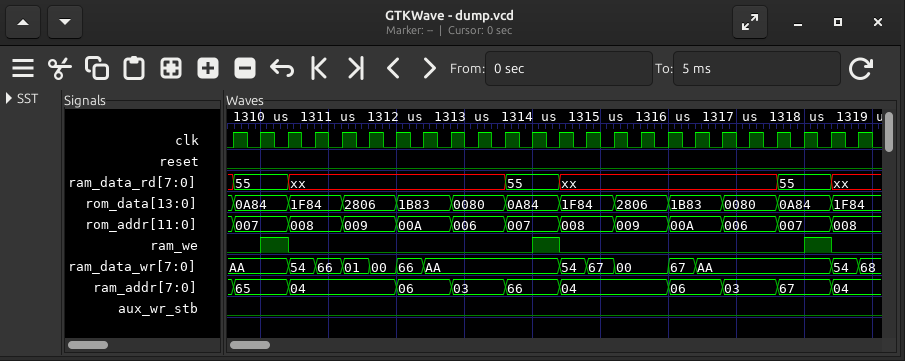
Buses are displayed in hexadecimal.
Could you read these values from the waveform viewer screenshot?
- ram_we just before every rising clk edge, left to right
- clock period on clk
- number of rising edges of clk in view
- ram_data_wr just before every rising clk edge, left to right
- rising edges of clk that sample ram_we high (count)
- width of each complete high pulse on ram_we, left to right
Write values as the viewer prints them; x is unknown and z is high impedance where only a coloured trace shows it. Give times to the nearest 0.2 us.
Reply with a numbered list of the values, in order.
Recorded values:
1. 0 0 1 0 0 0 0 0 0 0 0 0 1 0 0 0 0 0 0 0 0 0 1 0
2. 0.4 us
3. 24
4. AA, AA, AA, 54, 66, 01, 00, 66, AA, AA, AA, AA, AA, 54, 67, 00, 00, 67, AA, AA, AA, AA, AA, 54
5. 3
6. 0.4 us, 0.4 us, 0.4 us
